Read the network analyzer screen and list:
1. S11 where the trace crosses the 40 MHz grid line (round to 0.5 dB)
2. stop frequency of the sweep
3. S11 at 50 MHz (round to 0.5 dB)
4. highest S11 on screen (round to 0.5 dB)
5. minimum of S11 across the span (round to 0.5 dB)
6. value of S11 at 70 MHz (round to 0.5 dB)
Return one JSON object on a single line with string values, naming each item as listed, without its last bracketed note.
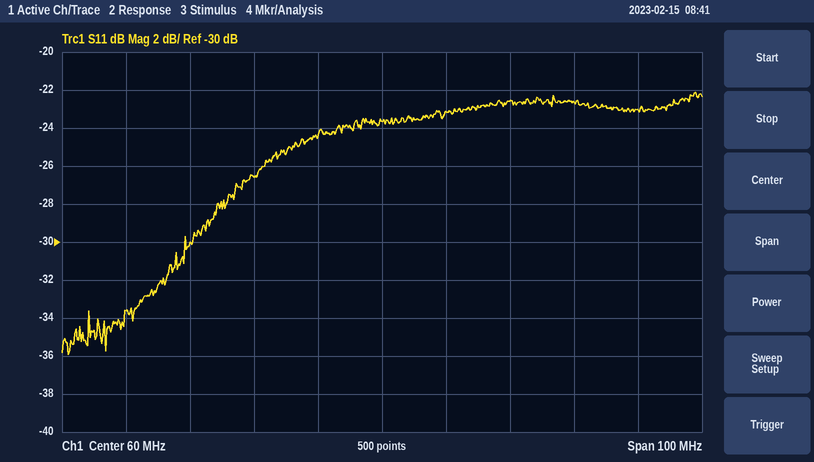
{"S11 where the trace crosses the 40 MHz grid line": "-26.5 dB", "stop frequency of the sweep": "110 MHz", "S11 at 50 MHz": "-24.5 dB", "highest S11 on screen": "-22.0 dB", "minimum of S11 across the span": "-36.0 dB", "value of S11 at 70 MHz": "-23.0 dB"}
